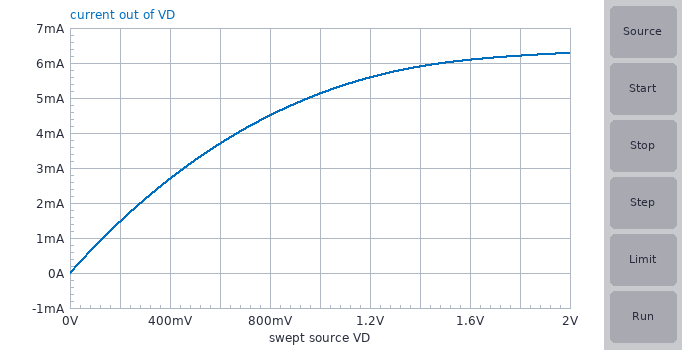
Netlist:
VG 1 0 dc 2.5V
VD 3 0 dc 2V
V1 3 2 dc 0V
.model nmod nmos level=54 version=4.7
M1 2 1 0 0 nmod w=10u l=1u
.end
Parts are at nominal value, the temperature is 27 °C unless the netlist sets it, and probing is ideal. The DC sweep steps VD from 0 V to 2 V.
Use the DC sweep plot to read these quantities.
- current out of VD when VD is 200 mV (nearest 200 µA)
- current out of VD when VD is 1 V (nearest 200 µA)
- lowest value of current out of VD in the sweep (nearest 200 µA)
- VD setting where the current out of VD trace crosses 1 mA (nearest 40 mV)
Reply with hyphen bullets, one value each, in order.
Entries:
- 1.4 mA
- 5.2 mA
- 0 A
- 120 mV
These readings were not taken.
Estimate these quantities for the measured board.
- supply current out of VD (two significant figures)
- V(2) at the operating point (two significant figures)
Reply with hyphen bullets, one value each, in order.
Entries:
- 6.3 mA
- 2.0 V
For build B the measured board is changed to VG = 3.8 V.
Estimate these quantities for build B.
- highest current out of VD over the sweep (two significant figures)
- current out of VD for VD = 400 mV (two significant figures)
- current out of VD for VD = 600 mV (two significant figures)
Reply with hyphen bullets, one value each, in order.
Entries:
- 11 mA
- 3.6 mA
- 5.0 mA
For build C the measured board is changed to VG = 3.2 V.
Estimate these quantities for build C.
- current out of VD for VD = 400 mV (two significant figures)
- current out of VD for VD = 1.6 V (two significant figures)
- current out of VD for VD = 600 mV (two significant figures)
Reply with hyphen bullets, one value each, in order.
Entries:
- 3.2 mA
- 8.2 mA
- 4.5 mA
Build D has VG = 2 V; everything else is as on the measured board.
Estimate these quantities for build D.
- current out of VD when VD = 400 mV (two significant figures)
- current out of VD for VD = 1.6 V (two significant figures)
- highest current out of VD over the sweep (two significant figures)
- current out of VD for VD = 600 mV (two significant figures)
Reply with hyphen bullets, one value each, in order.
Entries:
- 2.2 mA
- 4.4 mA
- 4.5 mA
- 3.0 mA
